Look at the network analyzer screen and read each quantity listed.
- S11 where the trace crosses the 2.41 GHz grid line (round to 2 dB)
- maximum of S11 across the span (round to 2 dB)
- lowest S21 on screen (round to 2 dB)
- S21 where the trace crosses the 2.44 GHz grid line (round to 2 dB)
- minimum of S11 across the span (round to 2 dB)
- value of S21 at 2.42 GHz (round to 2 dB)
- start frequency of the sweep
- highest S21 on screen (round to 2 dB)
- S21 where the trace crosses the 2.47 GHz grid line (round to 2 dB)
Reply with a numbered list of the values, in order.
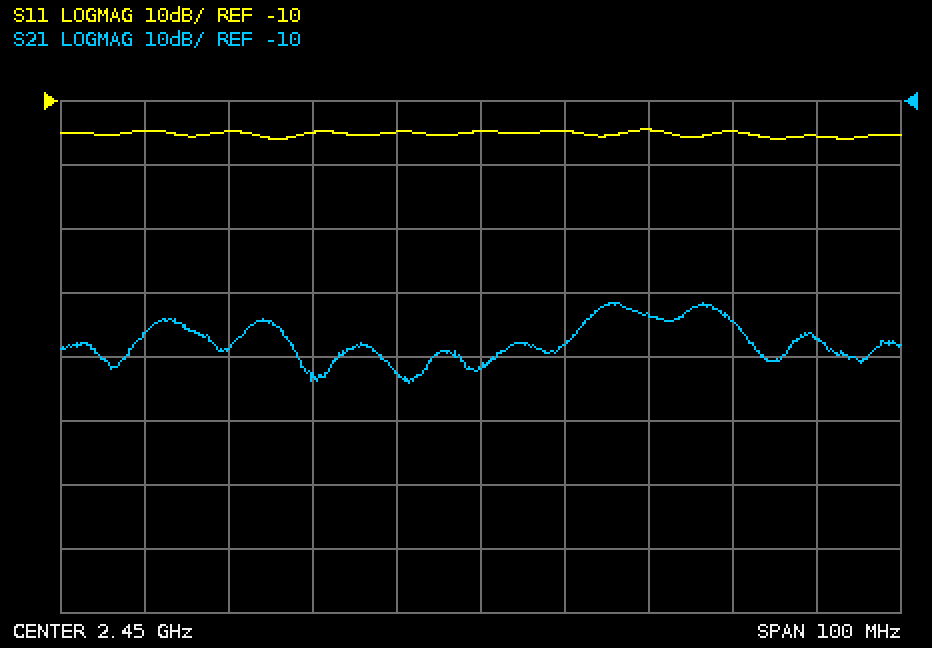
1. -14 dB
2. -14 dB
3. -54 dB
4. -52 dB
5. -16 dB
6. -48 dB
7. 2.4 GHz
8. -42 dB
9. -44 dB
